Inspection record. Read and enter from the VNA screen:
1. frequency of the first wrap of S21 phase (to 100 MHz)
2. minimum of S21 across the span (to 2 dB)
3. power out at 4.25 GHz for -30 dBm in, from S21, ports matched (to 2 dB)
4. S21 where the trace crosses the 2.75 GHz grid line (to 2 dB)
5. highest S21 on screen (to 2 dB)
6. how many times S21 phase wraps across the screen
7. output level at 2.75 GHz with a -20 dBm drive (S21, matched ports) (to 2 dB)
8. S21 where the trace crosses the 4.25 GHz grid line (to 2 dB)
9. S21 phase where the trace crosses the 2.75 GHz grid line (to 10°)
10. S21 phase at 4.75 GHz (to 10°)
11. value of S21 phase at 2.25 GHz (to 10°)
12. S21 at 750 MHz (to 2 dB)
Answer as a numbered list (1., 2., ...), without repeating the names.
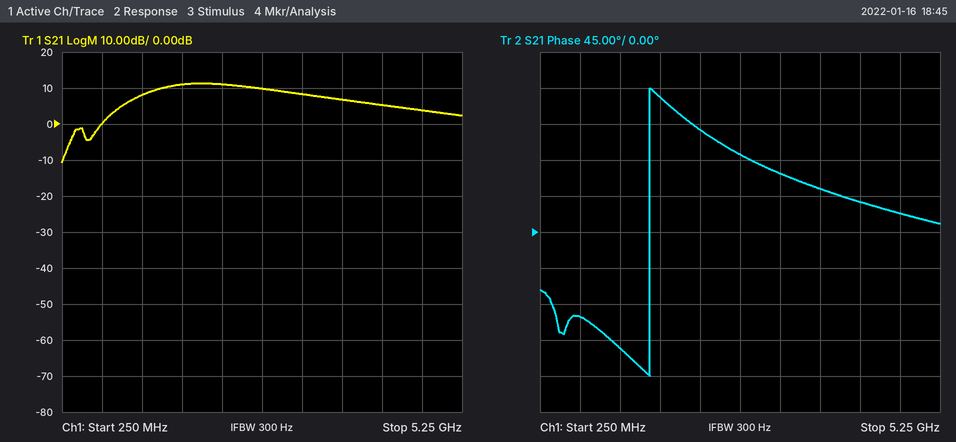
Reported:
1. 1.6 GHz
2. -10 dB
3. -24 dBm
4. 10 dB
5. 12 dB
6. 1
7. -10 dBm
8. 6 dB
9. 100°
10. 20°
11. 130°
12. 0 dB
